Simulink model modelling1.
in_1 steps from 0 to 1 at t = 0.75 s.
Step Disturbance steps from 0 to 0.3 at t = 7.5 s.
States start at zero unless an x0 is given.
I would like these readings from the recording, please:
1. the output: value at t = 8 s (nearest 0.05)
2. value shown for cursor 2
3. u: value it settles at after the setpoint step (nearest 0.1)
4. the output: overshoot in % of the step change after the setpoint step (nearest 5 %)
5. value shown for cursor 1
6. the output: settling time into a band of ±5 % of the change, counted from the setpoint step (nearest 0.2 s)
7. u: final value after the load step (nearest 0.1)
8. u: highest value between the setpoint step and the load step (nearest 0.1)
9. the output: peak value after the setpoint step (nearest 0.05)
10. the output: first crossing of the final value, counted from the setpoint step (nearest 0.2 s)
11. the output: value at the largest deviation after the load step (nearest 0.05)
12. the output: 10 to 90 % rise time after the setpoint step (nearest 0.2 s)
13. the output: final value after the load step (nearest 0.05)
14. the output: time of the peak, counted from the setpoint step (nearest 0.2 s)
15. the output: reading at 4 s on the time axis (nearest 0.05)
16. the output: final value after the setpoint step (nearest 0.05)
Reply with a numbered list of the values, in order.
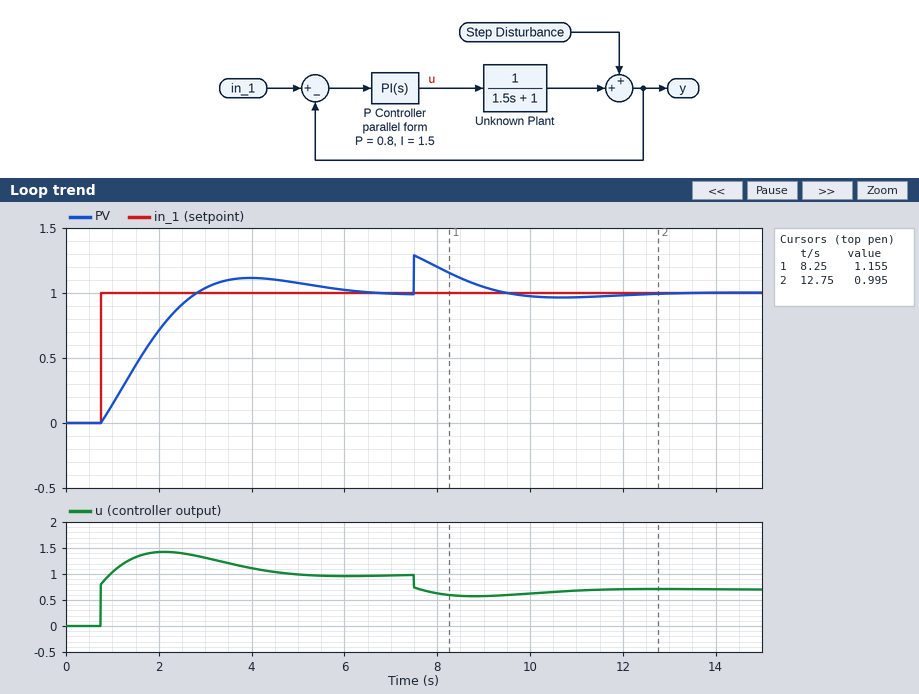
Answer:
1. 1.20
2. 0.995
3. 1.0
4. 10 %
5. 1.155
6. 4.8 s
7. 0.7
8. 1.4
9. 1.10
10. 2.0 s
11. 1.30
12. 1.6 s
13. 1.00
14. 3.2 s
15. 1.10
16. 1.00
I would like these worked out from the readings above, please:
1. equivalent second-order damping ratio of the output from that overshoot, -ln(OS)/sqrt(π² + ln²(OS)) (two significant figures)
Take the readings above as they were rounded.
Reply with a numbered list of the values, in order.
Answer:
1. 0.59
